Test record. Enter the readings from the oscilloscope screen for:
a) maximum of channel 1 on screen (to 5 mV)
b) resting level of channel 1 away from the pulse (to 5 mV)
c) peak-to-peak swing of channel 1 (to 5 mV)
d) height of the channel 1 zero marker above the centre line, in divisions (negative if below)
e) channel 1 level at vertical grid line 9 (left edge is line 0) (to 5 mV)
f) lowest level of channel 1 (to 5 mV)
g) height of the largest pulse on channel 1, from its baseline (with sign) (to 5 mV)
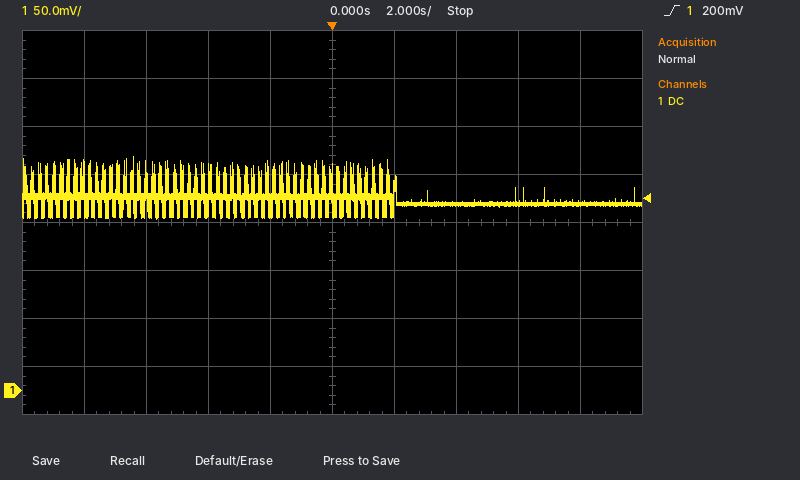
245 mV
195 mV
65 mV
-3.5 div
195 mV
180 mV
+50 mV
